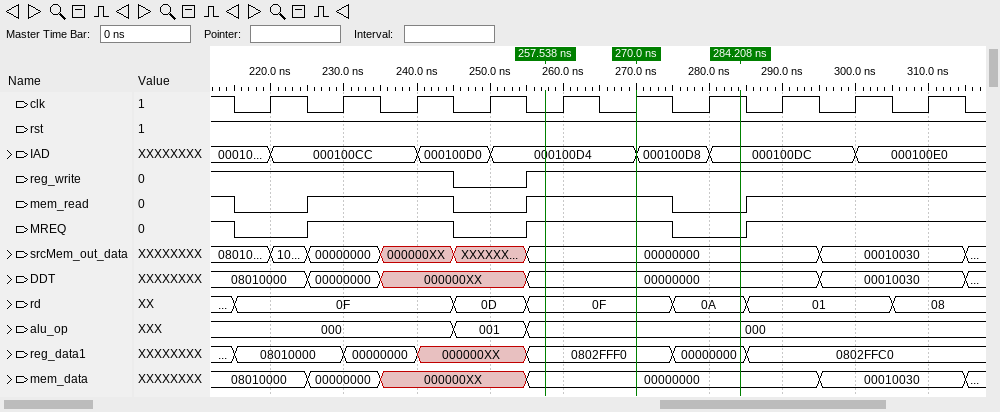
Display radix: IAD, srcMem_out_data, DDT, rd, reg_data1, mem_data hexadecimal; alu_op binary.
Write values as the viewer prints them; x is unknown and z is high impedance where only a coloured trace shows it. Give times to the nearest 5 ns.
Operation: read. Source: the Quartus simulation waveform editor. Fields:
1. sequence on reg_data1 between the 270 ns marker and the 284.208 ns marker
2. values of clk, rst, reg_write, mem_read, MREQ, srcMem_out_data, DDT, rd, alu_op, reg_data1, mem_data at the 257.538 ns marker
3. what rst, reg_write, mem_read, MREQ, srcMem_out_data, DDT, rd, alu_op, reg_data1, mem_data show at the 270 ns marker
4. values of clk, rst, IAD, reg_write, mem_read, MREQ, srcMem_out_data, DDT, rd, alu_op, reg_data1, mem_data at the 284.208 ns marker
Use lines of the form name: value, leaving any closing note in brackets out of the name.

sequence on reg_data1 between the 270 ns marker and the 284.208 ns marker: 0802FFF0, 00000000
values of clk, rst, reg_write, mem_read, MREQ, srcMem_out_data, DDT, rd, alu_op, reg_data1, mem_data at the 257.538 ns marker: clk=0, rst=1, reg_write=1, mem_read=1, MREQ=1, srcMem_out_data=00000000, DDT=00000000, rd=0F, alu_op=000, reg_data1=0802FFF0, mem_data=00000000
what rst, reg_write, mem_read, MREQ, srcMem_out_data, DDT, rd, alu_op, reg_data1, mem_data show at the 270 ns marker: rst=1, reg_write=1, mem_read=1, MREQ=1, srcMem_out_data=00000000, DDT=00000000, rd=0F, alu_op=000, reg_data1=0802FFF0, mem_data=00000000
values of clk, rst, IAD, reg_write, mem_read, MREQ, srcMem_out_data, DDT, rd, alu_op, reg_data1, mem_data at the 284.208 ns marker: clk=1, rst=1, IAD=000100DC, reg_write=1, mem_read=0, MREQ=0, srcMem_out_data=00000000, DDT=00000000, rd=0A, alu_op=000, reg_data1=00000000, mem_data=00000000
